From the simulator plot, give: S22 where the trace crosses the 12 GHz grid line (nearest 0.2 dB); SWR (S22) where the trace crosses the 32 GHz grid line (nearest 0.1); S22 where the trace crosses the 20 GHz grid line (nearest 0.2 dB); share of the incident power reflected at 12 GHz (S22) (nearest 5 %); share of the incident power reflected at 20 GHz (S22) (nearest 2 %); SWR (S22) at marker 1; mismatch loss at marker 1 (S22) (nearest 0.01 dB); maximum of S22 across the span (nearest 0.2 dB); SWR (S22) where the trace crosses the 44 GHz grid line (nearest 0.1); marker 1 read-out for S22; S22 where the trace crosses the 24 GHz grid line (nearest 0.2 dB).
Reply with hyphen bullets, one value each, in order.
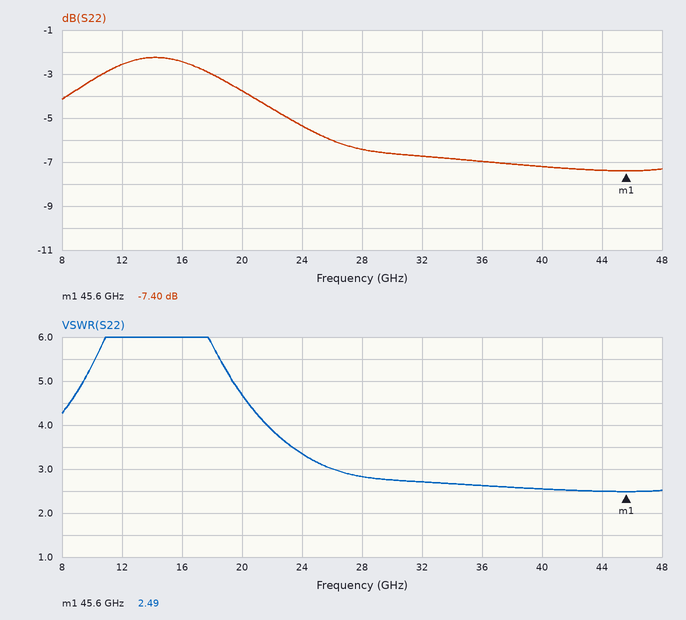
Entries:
- -2.6 dB
- 2.7
- -3.8 dB
- 55 %
- 42 %
- 2.49
- 0.87 dB
- -2.2 dB
- 2.5
- -7.40 dB
- -5.4 dB
